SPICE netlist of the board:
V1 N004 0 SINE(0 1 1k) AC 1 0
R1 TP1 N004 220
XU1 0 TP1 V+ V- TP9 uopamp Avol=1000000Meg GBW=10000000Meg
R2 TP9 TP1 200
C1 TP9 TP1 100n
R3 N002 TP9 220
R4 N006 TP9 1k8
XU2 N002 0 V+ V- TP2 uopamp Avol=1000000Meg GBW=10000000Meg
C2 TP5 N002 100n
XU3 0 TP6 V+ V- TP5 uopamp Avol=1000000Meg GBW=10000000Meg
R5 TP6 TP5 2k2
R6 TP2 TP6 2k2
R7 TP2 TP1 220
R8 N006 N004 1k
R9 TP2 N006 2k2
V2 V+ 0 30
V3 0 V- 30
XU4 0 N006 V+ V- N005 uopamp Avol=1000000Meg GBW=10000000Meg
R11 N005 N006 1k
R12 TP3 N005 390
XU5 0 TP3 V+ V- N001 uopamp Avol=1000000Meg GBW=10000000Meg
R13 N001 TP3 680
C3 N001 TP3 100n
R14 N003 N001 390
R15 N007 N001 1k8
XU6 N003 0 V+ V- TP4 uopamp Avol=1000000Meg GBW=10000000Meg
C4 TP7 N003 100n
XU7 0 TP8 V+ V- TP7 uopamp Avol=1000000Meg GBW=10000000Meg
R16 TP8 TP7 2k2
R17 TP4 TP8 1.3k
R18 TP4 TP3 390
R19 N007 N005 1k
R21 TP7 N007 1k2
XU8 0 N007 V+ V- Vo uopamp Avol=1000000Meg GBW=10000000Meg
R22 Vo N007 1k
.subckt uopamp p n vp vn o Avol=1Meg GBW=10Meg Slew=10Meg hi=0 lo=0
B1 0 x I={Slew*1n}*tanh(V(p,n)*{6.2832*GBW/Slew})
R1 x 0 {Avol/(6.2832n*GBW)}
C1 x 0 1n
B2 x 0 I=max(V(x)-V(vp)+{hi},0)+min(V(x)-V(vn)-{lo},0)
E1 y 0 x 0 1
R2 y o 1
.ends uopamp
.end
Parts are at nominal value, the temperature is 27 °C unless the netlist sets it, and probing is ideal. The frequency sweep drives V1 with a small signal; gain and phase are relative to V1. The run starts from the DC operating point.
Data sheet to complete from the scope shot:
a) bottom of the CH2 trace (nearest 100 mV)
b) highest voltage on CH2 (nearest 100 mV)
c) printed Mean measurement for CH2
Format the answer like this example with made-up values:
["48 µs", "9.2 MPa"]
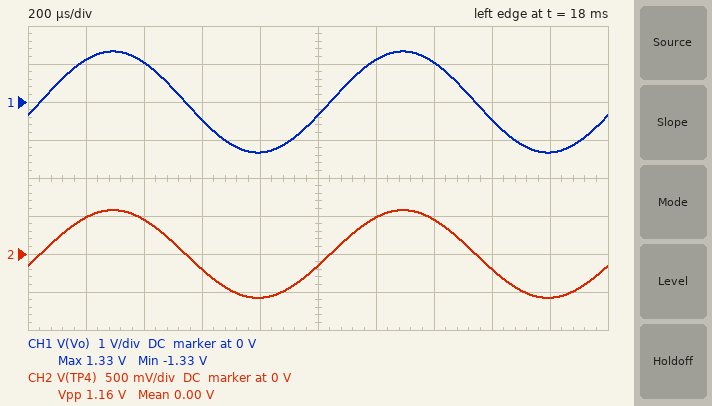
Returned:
["-600 mV", "600 mV", "0.00 V"]
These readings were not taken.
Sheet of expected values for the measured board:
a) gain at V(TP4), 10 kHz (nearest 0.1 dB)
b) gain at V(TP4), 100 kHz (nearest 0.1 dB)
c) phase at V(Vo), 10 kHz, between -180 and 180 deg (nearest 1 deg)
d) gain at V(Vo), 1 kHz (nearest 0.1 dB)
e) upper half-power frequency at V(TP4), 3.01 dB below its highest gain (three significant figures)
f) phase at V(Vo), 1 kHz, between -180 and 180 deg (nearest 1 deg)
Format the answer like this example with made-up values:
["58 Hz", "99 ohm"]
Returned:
["-20.6 dB", "-60.1 dB", "44 deg", "2.5 dB", "3.54 kHz", "-15 deg"]
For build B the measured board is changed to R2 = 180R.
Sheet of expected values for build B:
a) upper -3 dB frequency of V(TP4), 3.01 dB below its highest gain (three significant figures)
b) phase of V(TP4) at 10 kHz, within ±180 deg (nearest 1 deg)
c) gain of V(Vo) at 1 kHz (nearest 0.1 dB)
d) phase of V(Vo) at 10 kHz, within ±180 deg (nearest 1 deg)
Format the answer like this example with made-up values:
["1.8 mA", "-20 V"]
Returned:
["3.61 kHz", "-138 deg", "2.5 dB", "42 deg"]
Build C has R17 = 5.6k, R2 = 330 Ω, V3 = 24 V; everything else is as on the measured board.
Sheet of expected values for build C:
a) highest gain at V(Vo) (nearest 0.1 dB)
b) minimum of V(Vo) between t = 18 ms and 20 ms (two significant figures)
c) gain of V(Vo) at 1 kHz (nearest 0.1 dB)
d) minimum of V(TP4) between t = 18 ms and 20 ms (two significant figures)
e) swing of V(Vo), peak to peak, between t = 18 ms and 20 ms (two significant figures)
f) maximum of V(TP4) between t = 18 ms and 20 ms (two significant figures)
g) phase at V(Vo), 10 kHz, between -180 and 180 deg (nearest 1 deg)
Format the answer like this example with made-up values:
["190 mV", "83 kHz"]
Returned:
["0 dB", "-710 mV", "-2.9 dB", "-550 mV", "1.4 V", "550 mV", "60 deg"]
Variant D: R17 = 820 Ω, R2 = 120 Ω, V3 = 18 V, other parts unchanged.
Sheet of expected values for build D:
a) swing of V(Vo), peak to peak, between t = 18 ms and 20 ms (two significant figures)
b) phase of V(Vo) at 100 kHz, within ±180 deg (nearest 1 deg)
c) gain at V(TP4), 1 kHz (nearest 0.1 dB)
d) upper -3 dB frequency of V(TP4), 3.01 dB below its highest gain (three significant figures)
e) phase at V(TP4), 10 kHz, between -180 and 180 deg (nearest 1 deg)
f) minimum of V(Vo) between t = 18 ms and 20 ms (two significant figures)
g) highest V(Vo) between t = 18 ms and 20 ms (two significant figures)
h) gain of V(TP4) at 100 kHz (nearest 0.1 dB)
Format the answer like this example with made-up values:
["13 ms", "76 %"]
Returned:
["3.7 V", "4 deg", "-4.5 dB", "3.00 kHz", "-148 deg", "-1.8 V", "1.8 V", "-64.2 dB"]
